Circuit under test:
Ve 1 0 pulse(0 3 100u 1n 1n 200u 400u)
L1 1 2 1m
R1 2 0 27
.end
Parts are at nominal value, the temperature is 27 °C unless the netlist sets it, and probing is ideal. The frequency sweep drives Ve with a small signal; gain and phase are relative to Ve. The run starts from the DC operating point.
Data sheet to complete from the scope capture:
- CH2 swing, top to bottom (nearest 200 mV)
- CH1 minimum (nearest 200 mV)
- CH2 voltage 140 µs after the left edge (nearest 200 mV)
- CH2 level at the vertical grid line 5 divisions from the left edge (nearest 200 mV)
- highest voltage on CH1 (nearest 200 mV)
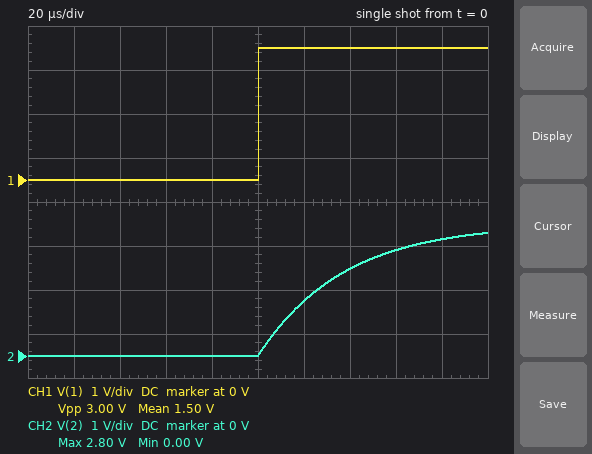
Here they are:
2.8 V
0 V
2.0 V
0 V
3.0 V
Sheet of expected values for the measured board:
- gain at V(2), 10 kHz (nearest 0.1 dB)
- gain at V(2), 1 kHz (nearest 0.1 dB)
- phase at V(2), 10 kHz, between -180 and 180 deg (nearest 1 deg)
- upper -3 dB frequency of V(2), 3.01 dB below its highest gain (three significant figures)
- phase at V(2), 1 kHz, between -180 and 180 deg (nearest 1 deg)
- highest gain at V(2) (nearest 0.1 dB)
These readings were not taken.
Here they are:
-8.1 dB
-0.2 dB
-67 deg
4.30 kHz
-13 deg
0 dB
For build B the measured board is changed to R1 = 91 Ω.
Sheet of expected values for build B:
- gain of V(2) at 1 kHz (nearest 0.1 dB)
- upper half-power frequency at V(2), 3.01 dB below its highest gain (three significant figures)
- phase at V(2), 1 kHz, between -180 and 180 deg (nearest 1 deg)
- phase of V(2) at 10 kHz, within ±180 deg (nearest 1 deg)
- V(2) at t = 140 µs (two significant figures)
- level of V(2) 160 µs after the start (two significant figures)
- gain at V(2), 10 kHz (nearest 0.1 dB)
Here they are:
0 dB
14.5 kHz
-4 deg
-35 deg
2.9 V
3.0 V
-1.7 dB
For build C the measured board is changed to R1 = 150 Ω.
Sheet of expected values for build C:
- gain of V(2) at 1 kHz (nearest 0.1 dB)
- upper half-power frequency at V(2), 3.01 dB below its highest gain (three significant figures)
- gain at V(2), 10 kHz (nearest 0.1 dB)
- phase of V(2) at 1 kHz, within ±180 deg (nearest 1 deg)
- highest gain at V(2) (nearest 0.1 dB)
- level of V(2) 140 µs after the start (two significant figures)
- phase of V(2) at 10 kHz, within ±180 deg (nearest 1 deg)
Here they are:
0 dB
23.9 kHz
-0.7 dB
-2 deg
0 dB
3.0 V
-23 deg
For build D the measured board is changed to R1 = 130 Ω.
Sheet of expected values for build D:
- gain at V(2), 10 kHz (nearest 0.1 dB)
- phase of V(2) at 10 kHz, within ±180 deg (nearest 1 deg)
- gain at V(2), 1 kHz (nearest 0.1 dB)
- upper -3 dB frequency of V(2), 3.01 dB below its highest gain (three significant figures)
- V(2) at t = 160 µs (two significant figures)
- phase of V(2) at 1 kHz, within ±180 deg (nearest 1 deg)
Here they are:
-0.9 dB
-26 deg
0 dB
20.7 kHz
3.0 V
-3 deg
